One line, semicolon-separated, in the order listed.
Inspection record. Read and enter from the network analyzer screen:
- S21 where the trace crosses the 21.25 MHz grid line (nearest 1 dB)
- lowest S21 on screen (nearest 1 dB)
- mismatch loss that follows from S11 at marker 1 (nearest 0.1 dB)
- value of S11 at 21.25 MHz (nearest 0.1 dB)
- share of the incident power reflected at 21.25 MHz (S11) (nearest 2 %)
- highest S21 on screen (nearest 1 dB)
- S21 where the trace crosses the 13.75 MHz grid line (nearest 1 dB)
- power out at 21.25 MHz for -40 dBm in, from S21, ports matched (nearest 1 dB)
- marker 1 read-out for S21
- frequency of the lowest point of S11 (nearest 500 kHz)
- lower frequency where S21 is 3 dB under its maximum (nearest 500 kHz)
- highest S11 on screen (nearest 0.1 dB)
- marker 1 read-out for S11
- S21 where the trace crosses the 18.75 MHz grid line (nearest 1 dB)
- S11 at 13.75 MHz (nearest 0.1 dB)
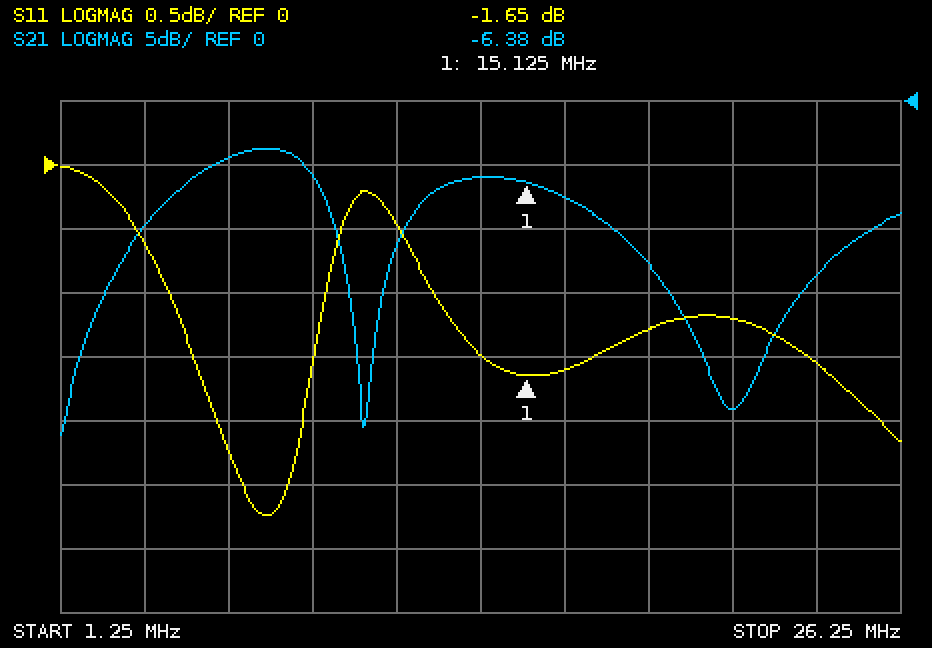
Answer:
-24 dB; -26 dB; 5.0 dB; -1.2 dB; 76 %; -4 dB; -6 dB; -64 dBm; -6.38 dB; 7.5 MHz; 5.0 MHz; 0.0 dB; -1.65 dB; -13 dB; -1.5 dB
